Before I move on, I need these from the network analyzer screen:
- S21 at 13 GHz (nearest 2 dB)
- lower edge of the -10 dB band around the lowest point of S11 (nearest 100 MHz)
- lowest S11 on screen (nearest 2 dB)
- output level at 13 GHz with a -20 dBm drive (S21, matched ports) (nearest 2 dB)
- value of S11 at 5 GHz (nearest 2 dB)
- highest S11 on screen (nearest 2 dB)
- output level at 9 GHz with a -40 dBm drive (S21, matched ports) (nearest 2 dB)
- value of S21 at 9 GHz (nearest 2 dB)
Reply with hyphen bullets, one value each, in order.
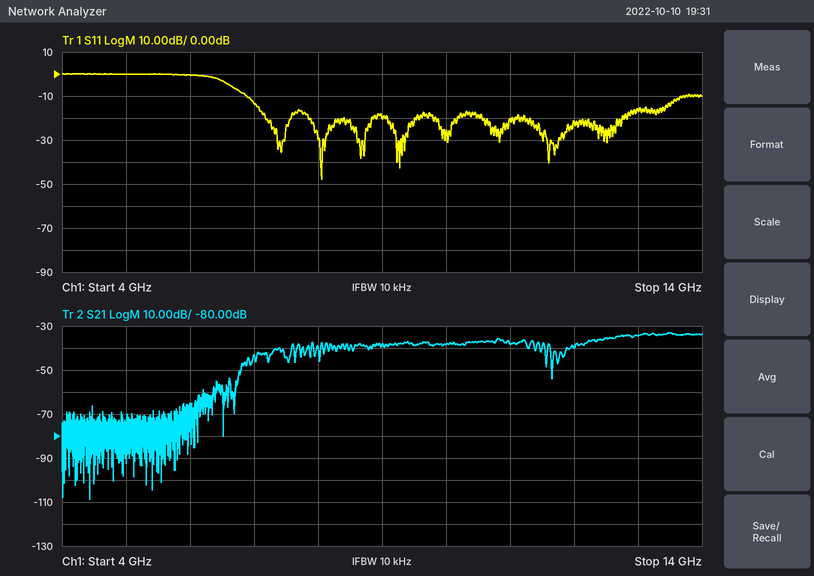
- -34 dB
- 6.9 GHz
- -48 dB
- -54 dBm
- 0 dB
- 0 dB
- -78 dBm
- -38 dB
